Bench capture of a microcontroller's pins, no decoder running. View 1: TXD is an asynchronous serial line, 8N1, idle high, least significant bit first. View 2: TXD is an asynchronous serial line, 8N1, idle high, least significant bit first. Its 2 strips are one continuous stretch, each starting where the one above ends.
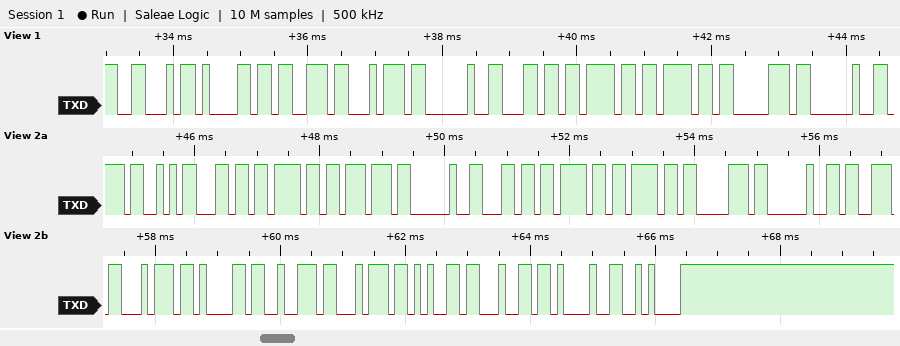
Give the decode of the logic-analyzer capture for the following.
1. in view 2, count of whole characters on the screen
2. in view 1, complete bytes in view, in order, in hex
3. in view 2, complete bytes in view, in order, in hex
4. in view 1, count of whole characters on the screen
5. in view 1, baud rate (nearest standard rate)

19
46 61 73 74 20 6C 6F 6F 70 20
0x53 0x6C 0x6F 0x77 0x20 0x6C 0x6F 0x6F 0x70 0x20 0x73 0x74 0x61 0x72 0x74 0x65 0x64 0x21 0x0A
10
9600 baud
